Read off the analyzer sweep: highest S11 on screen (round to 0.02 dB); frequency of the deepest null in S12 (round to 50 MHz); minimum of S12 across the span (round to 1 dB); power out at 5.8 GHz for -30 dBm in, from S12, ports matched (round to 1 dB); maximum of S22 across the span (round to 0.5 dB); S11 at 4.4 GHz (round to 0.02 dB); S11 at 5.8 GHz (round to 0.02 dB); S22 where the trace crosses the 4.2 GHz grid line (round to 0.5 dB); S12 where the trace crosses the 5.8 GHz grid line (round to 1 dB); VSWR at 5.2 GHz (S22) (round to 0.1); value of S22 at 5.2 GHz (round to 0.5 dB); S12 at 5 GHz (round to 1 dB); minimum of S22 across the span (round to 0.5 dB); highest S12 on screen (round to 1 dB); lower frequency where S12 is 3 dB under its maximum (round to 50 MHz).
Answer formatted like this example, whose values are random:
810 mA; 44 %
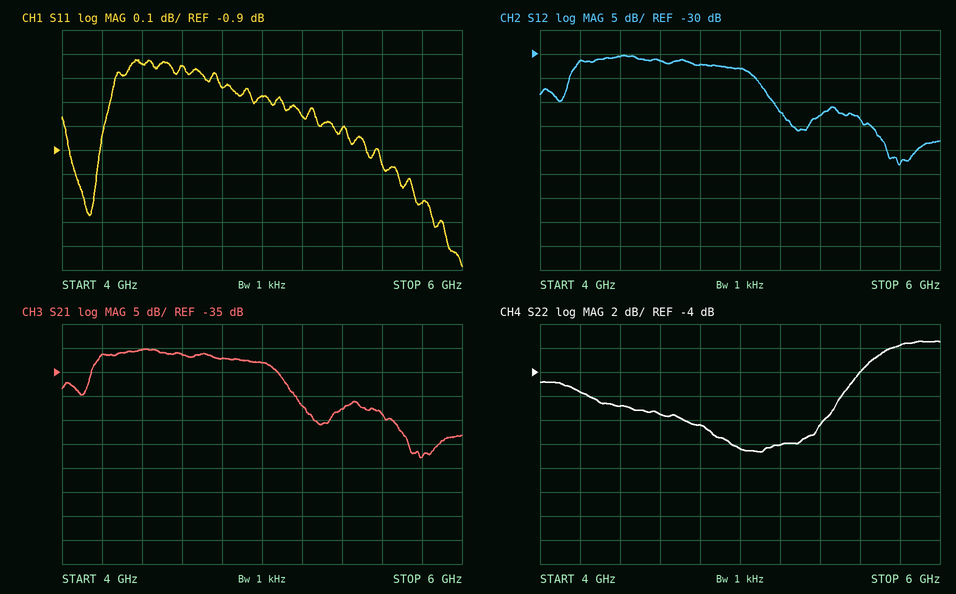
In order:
-0.52 dB; 5.80 GHz; -53 dB; -83 dBm; -1.5 dB; -0.54 dB; -1.12 dB; -5.5 dB; -53 dB; 1.9; -10.0 dB; -33 dB; -10.5 dB; -30 dB; 4.15 GHz
